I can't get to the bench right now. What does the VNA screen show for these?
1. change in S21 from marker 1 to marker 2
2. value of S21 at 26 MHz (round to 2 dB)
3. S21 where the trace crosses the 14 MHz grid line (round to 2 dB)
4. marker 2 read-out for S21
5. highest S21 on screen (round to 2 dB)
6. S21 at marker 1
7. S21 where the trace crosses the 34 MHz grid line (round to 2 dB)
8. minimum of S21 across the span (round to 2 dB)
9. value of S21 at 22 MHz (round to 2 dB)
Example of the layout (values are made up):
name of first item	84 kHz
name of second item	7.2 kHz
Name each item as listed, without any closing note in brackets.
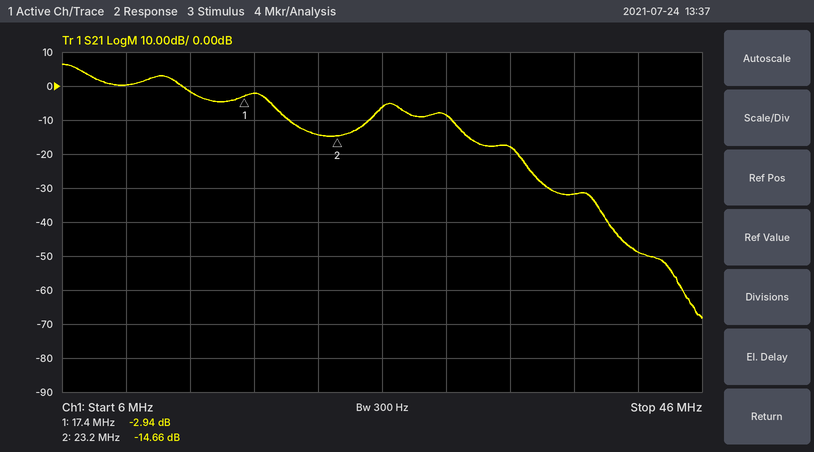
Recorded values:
change in S21 from marker 1 to marker 2	-11.72 dB
value of S21 at 26 MHz	-6 dB
S21 where the trace crosses the 14 MHz grid line	-2 dB
marker 2 read-out for S21	-14.66 dB
highest S21 on screen	6 dB
S21 at marker 1	-2.94 dB
S21 where the trace crosses the 34 MHz grid line	-18 dB
minimum of S21 across the span	-68 dB
value of S21 at 22 MHz	-14 dB
